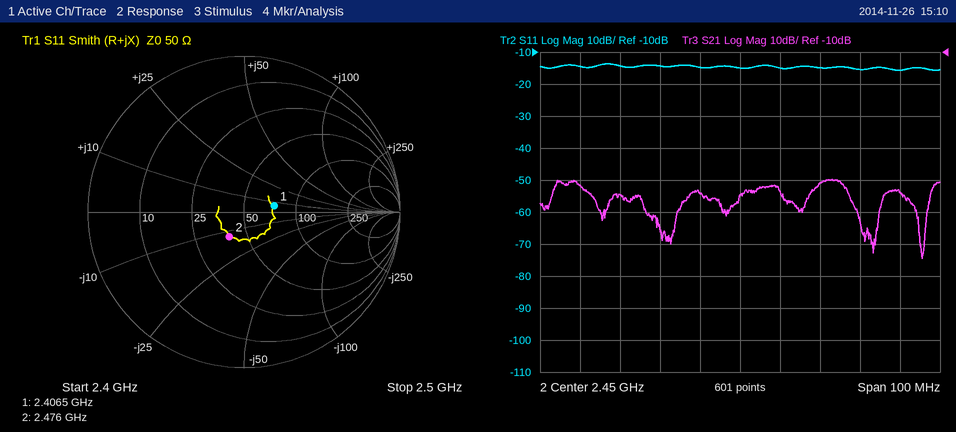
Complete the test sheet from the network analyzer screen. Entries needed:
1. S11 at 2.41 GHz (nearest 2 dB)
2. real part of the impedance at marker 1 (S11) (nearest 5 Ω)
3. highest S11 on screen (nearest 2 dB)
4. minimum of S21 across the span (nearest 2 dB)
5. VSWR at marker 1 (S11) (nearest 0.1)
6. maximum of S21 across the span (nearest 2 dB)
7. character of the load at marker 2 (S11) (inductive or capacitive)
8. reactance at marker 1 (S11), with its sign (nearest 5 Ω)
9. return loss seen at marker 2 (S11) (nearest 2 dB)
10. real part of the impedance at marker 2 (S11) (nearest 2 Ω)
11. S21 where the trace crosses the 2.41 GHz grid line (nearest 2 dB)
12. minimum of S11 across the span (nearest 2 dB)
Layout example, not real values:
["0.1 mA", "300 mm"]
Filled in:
["-14 dB", "75 Ω", "-14 dB", "-74 dB", "1.5", "-50 dB", "capacitive", "+5 Ω", "14 dB", "40 Ω", "-52 dB", "-16 dB"]
